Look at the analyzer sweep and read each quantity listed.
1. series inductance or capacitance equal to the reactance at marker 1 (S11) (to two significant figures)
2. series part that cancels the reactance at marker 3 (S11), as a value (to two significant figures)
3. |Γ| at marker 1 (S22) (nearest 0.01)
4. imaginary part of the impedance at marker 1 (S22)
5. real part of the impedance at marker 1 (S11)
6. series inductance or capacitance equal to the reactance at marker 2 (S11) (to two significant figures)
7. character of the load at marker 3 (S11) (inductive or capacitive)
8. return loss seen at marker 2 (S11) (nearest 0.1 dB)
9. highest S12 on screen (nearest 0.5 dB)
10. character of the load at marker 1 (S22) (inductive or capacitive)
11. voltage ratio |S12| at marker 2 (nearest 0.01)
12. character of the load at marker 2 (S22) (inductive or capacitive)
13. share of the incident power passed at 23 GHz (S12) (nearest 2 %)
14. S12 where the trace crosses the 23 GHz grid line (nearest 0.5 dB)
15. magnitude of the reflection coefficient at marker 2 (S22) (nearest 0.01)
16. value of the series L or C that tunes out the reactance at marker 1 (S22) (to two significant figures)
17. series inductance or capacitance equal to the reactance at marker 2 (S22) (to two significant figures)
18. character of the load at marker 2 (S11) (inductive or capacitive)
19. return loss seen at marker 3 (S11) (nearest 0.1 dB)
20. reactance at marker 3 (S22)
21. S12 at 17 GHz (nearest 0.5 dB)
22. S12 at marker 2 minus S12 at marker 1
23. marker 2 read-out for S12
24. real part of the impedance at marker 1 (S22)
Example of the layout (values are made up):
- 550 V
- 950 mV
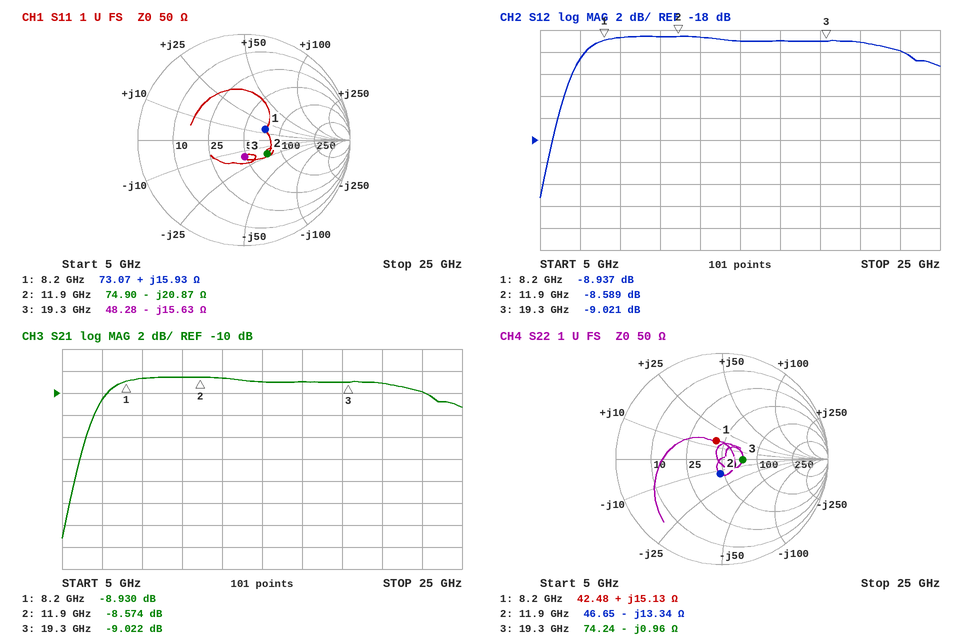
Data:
- 310 pH
- 130 pH
- 0.18
- +15.13 Ω
- 73.07 Ω
- 640 fF
- capacitive
- 11.8 dB
- -8.5 dB
- inductive
- 0.37
- capacitive
- 10 %
- -10.0 dB
- 0.14
- 1.3 pF
- 1.0 pF
- capacitive
- 16.0 dB
- -0.96 Ω
- -9.0 dB
- 0.348 dB
- -8.589 dB
- 42.48 Ω
